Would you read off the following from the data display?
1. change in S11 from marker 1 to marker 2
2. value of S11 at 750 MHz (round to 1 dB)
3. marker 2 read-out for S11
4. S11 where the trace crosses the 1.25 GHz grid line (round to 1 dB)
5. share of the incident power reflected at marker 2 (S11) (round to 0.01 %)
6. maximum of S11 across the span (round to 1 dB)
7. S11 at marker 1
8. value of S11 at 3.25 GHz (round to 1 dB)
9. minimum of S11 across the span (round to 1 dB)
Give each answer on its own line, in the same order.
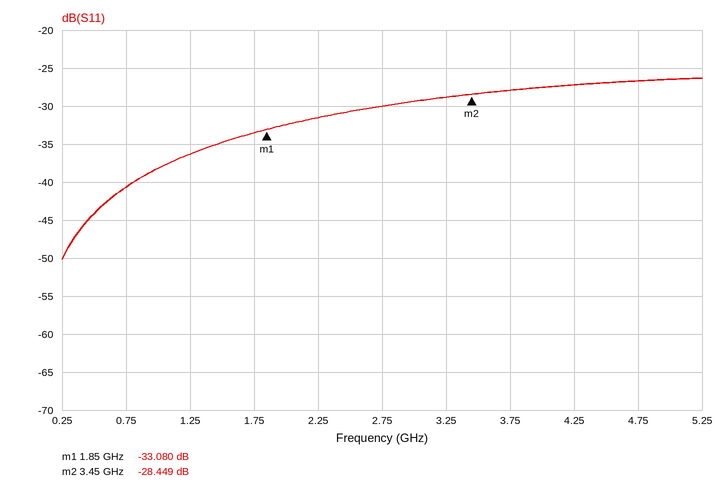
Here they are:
4.631 dB
-41 dB
-28.449 dB
-36 dB
0.14 %
-26 dB
-33.080 dB
-29 dB
-50 dB
